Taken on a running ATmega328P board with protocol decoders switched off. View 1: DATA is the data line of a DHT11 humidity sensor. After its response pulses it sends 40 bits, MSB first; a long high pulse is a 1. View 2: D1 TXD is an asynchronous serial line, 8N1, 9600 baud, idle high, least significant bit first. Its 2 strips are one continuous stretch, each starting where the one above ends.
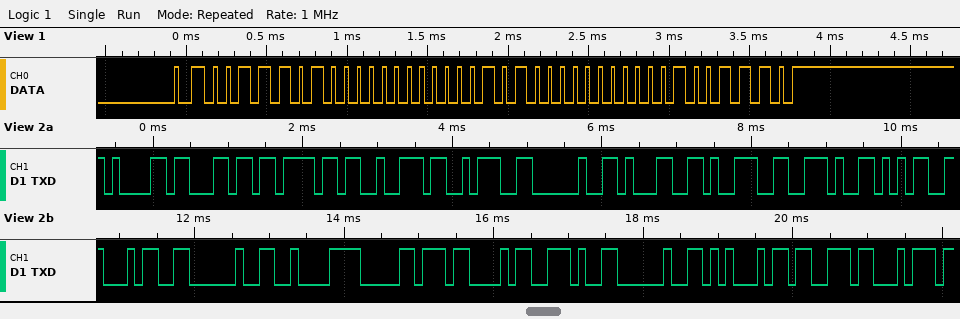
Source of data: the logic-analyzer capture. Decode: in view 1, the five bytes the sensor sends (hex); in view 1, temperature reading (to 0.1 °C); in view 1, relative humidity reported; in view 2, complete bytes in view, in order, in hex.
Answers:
3A 00 14 00 4E
20.0 °C
58 %
61 6C 6F 72 3A 20 31 39 2E 35 34 20 C2 B0 43 2E 20 45 73 74
